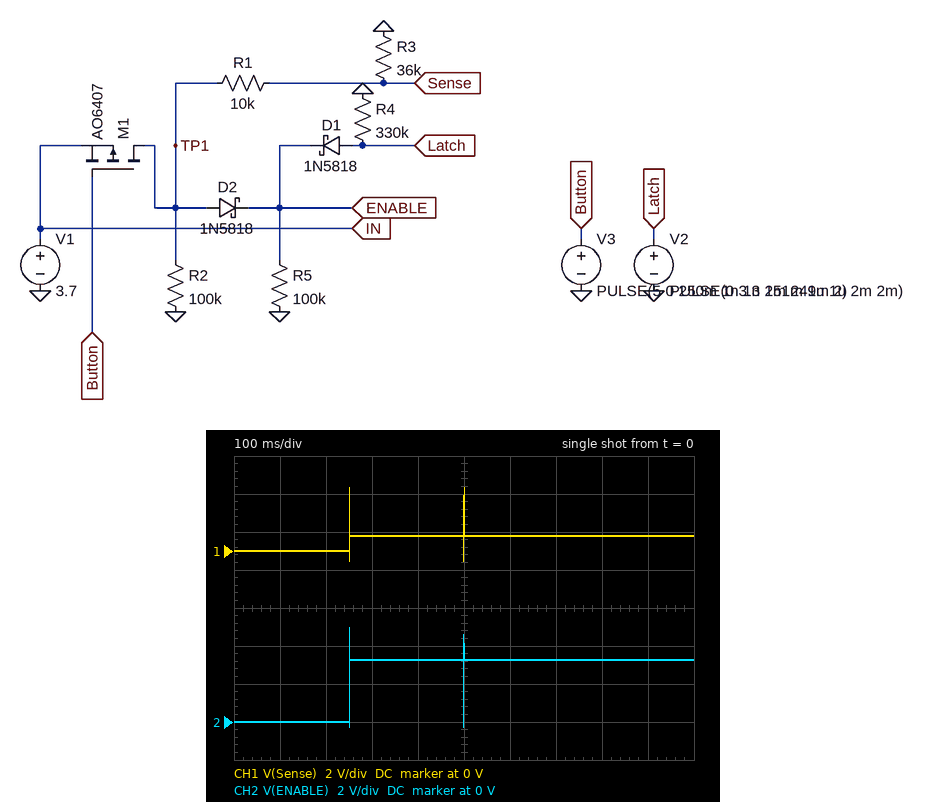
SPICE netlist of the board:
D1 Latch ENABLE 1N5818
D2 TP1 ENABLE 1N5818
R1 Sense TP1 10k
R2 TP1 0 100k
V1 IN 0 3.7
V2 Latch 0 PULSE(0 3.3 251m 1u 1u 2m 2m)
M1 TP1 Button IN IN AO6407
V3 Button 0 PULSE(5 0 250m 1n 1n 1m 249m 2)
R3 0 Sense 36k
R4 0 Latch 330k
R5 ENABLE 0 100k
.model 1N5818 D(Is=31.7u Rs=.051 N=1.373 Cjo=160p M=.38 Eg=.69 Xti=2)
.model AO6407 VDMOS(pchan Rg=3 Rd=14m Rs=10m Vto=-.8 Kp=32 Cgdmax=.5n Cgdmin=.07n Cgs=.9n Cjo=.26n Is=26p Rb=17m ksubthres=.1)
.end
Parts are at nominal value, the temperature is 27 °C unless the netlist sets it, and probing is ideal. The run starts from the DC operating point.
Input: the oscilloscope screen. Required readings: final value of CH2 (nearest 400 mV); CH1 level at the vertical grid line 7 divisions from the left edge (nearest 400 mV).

3.2 V
800 mV
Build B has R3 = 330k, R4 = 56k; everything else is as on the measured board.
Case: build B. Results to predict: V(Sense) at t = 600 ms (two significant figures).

2.4 V
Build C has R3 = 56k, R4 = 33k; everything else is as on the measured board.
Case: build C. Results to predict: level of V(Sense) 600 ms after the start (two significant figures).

1.1 V
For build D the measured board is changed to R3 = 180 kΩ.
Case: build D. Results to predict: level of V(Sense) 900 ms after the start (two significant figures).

2.0 V
